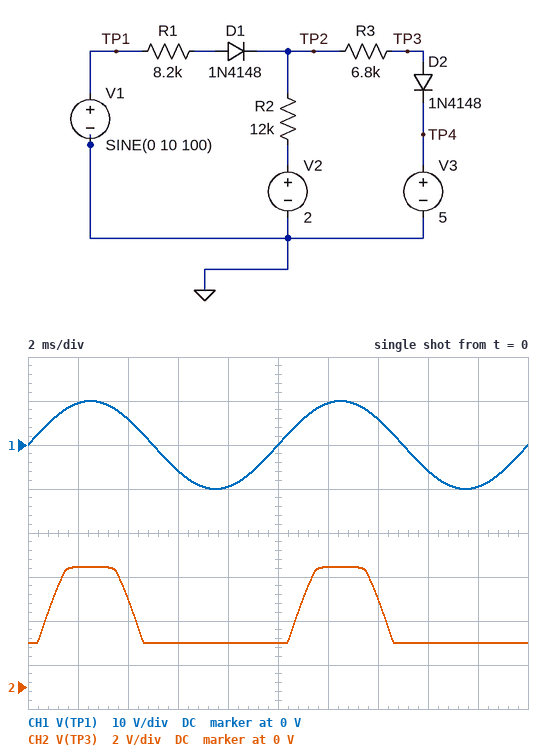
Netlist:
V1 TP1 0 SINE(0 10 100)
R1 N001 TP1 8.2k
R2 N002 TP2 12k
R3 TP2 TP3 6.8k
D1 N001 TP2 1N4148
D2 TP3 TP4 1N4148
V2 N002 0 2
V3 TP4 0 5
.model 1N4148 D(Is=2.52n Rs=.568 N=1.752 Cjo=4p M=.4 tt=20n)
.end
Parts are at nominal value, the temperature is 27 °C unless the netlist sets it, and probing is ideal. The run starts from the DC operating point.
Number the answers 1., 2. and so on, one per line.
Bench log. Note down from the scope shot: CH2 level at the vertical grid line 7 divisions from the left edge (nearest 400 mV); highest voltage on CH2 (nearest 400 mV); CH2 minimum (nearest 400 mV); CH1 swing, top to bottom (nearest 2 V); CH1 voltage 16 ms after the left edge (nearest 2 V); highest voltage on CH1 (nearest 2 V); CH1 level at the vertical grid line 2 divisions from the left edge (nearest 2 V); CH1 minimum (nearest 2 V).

1. 4.0 V
2. 5.6 V
3. 2.0 V
4. 20 V
5. -6 V
6. 10 V
7. 6 V
8. -10 V
